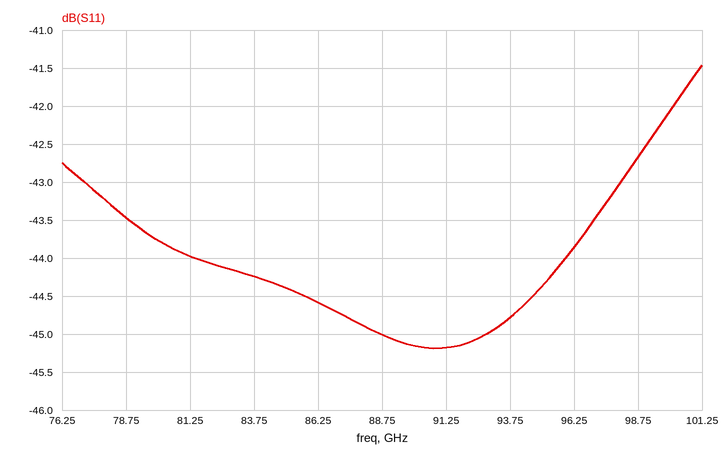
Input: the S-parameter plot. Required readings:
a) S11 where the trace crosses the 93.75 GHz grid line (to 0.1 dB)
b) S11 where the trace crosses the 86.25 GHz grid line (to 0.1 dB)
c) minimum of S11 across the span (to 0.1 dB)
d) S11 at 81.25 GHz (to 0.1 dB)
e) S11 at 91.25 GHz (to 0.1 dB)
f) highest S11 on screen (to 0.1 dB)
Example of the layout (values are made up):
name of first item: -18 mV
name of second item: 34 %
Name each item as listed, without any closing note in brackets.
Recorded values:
S11 where the trace crosses the 93.75 GHz grid line: -44.8 dB
S11 where the trace crosses the 86.25 GHz grid line: -44.6 dB
minimum of S11 across the span: -45.2 dB
S11 at 81.25 GHz: -44.0 dB
S11 at 91.25 GHz: -45.2 dB
highest S11 on screen: -41.5 dB
